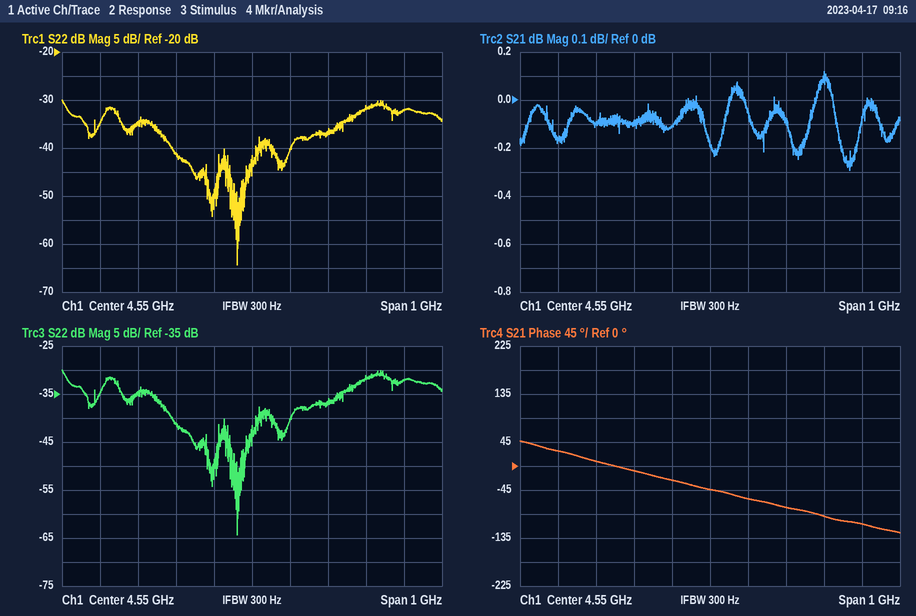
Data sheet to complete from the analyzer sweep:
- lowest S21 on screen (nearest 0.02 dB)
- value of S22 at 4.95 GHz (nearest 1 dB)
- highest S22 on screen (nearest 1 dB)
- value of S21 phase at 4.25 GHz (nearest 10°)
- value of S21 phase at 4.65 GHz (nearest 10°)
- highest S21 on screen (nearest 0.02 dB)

-0.30 dB
-32 dB
-30 dB
10°
-60°
0.12 dB
